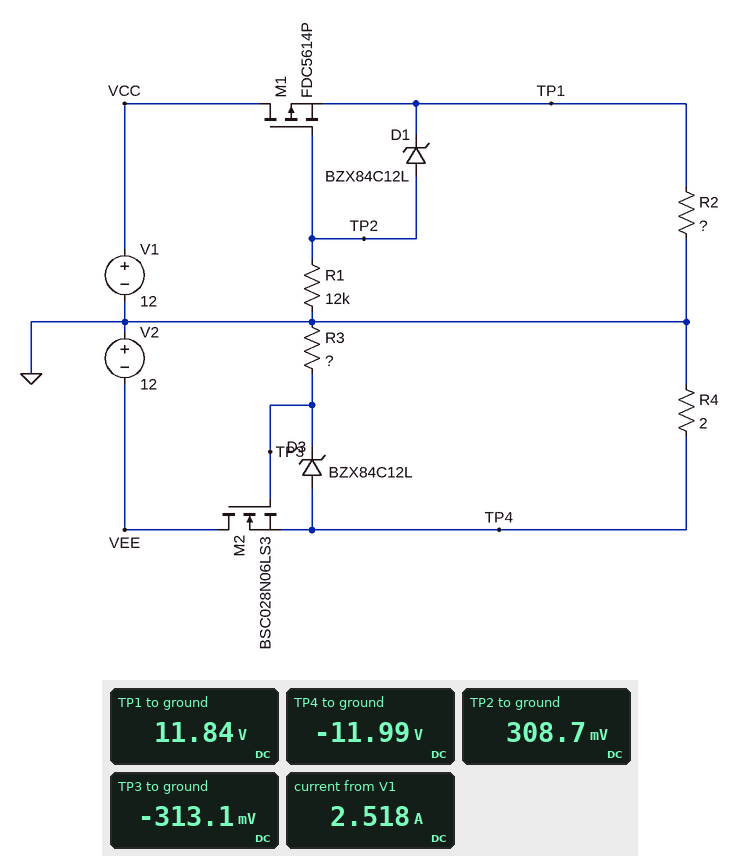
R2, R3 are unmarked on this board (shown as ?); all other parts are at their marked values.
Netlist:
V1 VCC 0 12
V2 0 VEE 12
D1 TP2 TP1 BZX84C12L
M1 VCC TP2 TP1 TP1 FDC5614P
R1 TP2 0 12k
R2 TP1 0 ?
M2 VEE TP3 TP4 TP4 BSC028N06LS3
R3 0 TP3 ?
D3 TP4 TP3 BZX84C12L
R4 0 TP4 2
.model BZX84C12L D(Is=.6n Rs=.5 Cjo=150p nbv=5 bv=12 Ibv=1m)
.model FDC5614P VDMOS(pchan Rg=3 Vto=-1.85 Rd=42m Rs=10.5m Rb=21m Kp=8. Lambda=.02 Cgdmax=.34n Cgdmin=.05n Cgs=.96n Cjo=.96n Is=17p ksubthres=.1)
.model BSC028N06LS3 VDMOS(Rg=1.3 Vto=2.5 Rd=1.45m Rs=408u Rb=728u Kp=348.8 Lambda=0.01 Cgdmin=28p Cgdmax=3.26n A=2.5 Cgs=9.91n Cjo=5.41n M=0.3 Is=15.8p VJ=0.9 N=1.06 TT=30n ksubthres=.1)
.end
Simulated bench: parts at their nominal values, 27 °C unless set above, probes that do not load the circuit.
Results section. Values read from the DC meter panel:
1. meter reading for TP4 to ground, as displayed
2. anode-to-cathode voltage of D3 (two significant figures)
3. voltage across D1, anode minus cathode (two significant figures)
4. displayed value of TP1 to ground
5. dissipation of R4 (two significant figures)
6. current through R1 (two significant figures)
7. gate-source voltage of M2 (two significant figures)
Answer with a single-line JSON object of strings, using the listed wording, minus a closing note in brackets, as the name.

{"meter reading for TP4 to ground, as displayed": "-11.99 V", "anode-to-cathode voltage of D3": "-12 V", "voltage across D1, anode minus cathode": "-12 V", "displayed value of TP1 to ground": "11.84 V", "dissipation of R4": "72 W", "current through R1": "26 µA", "gate-source voltage of M2": "12 V"}
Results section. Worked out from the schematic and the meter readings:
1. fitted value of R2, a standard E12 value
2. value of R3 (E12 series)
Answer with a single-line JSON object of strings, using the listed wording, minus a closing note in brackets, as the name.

{"fitted value of R2, a standard E12 value": "4.7 Ω", "value of R3": "3.9 kΩ"}
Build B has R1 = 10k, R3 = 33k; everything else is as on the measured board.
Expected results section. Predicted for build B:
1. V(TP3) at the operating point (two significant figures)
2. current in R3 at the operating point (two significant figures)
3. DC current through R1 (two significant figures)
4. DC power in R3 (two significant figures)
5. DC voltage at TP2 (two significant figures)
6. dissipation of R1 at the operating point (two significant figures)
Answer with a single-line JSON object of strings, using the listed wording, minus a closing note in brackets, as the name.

{"V(TP3) at the operating point": "-520 mV", "current in R3 at the operating point": "16 µA", "DC current through R1": "29 µA", "DC power in R3": "8.3 µW", "DC voltage at TP2": "290 mV", "dissipation of R1 at the operating point": "8.5 µW"}
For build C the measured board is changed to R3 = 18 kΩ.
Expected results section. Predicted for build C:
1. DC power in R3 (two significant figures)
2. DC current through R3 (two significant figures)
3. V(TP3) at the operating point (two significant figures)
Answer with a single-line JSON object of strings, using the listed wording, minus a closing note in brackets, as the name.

{"DC power in R3": "12 µW", "DC current through R3": "26 µA", "V(TP3) at the operating point": "-460 mV"}
